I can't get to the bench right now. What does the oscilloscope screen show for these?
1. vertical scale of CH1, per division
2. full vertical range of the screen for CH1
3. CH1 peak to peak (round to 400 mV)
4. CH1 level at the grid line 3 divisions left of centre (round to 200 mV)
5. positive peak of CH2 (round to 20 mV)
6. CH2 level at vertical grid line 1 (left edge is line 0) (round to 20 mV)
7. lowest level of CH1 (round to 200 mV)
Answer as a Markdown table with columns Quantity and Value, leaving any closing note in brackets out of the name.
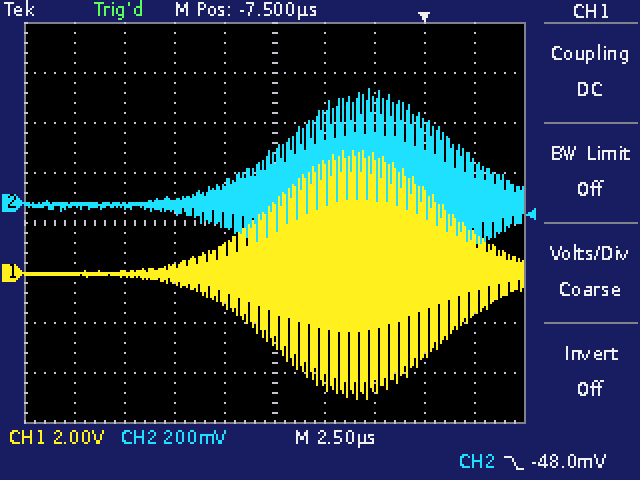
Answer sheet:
| Quantity | Value |
|---|---|
| vertical scale of CH1, per division | 2 V |
| full vertical range of the screen for CH1 | 16 V |
| CH1 peak to peak | 10.0 V |
| CH1 level at the grid line 3 divisions left of centre | 0.0 V |
| positive peak of CH2 | 460 mV |
| CH2 level at vertical grid line 1 (left edge is line 0) | 0 mV |
| lowest level of CH1 | -5.0 V |
